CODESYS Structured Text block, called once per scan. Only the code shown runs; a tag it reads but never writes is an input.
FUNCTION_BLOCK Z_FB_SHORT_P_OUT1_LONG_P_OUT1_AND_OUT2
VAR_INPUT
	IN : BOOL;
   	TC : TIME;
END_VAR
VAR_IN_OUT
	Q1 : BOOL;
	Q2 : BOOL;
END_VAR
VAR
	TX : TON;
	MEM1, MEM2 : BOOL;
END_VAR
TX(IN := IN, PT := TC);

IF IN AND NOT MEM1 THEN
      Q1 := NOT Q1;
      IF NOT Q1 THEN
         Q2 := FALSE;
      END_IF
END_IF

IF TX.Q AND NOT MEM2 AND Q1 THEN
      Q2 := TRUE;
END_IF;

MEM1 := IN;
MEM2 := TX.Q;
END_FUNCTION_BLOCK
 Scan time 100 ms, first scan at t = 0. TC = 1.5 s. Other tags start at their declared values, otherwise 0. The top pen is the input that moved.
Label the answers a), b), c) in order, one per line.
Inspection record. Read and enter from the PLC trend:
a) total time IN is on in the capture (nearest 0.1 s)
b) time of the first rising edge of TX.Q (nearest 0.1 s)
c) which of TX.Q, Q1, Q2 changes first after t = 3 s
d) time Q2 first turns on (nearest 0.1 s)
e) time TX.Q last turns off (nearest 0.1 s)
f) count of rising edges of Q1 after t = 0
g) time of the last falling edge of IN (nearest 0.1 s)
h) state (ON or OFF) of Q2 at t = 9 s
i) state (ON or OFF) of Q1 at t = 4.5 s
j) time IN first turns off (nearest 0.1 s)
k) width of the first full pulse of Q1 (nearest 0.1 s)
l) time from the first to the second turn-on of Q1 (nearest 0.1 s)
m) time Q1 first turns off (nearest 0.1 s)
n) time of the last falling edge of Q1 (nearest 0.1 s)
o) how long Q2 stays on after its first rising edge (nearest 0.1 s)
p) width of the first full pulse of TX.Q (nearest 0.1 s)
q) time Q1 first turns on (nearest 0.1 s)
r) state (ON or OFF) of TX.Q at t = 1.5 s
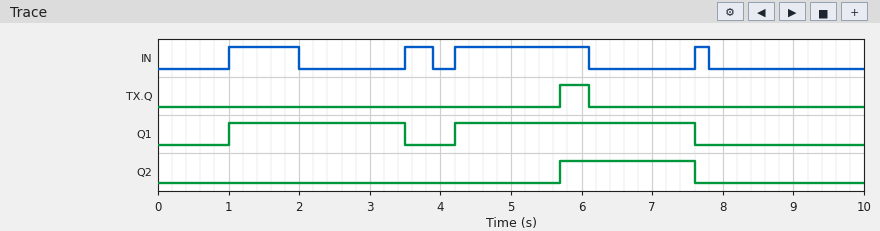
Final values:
a) 3.5 s
b) 5.7 s
c) Q1
d) 5.7 s
e) 6.1 s
f) 2
g) 7.8 s
h) OFF
i) ON
j) 2.0 s
k) 2.5 s
l) 3.2 s
m) 3.5 s
n) 7.6 s
o) 1.9 s
p) 0.4 s
q) 1.0 s
r) OFF
